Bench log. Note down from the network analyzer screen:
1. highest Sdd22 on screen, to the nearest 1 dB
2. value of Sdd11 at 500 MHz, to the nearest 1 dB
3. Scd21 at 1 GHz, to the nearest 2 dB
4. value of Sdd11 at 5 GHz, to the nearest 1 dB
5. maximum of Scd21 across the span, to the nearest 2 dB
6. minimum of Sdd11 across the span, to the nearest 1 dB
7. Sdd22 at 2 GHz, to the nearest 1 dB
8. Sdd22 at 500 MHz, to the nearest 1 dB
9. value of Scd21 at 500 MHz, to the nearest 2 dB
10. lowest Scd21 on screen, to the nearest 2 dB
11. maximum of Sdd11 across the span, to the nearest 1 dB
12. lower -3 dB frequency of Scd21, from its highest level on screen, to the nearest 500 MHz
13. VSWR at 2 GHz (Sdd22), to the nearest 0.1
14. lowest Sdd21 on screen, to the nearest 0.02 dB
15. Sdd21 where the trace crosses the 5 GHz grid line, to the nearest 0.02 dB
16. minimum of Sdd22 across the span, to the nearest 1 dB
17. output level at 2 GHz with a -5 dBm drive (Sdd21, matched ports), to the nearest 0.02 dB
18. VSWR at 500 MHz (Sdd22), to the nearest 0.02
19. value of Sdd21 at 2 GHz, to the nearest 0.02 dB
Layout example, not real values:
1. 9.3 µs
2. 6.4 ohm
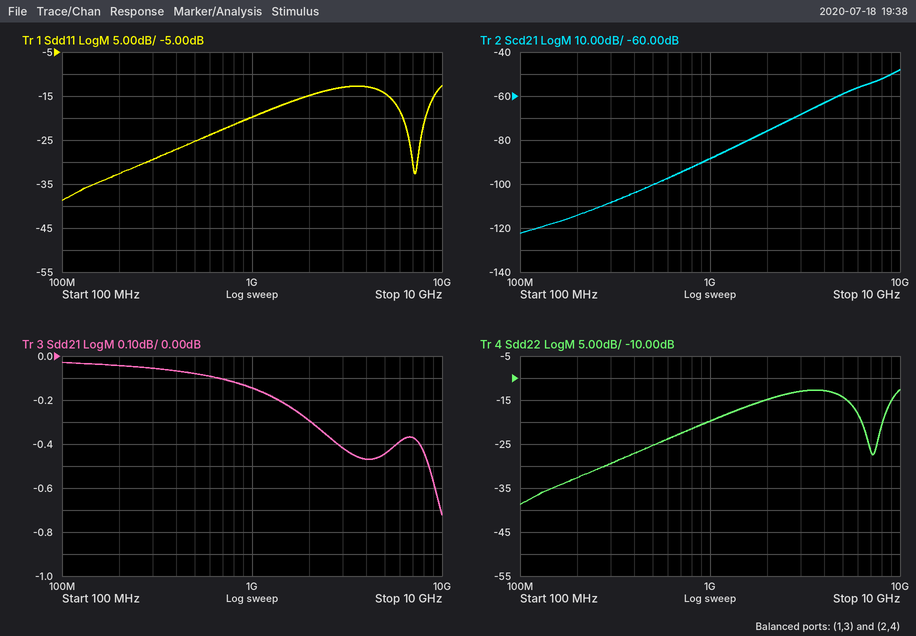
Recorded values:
1. -13 dB
2. -25 dB
3. -88 dB
4. -14 dB
5. -48 dB
6. -39 dB
7. -15 dB
8. -25 dB
9. -100 dB
10. -122 dB
11. -13 dB
12. 8.5 GHz
13. 1.4
14. -0.72 dB
15. -0.44 dB
16. -39 dB
17. -5.30 dBm
18. 1.12
19. -0.30 dB
